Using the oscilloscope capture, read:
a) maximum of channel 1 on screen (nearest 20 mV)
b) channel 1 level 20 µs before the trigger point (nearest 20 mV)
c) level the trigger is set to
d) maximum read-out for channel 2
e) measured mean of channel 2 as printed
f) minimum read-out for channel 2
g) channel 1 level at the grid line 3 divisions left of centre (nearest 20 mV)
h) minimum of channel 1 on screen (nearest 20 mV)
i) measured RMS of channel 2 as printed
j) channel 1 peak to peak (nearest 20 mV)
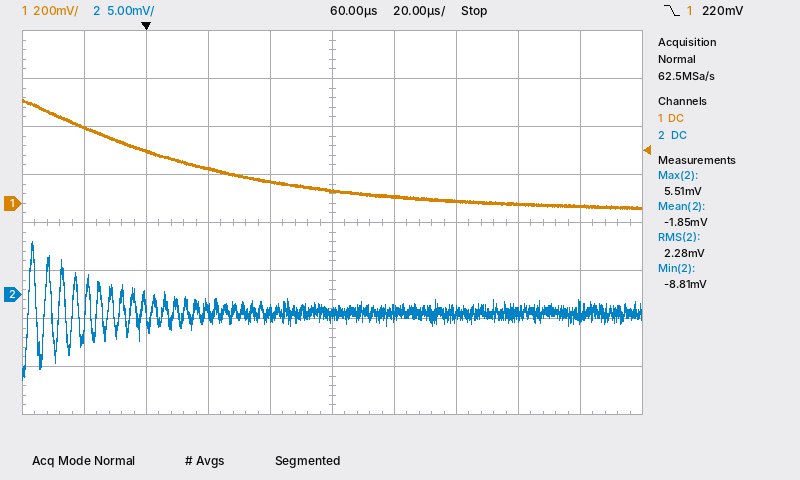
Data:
440 mV
320 mV
220 mV
5.51 mV
-1.85 mV
-8.81 mV
220 mV
-20 mV
2.28 mV
460 mV
